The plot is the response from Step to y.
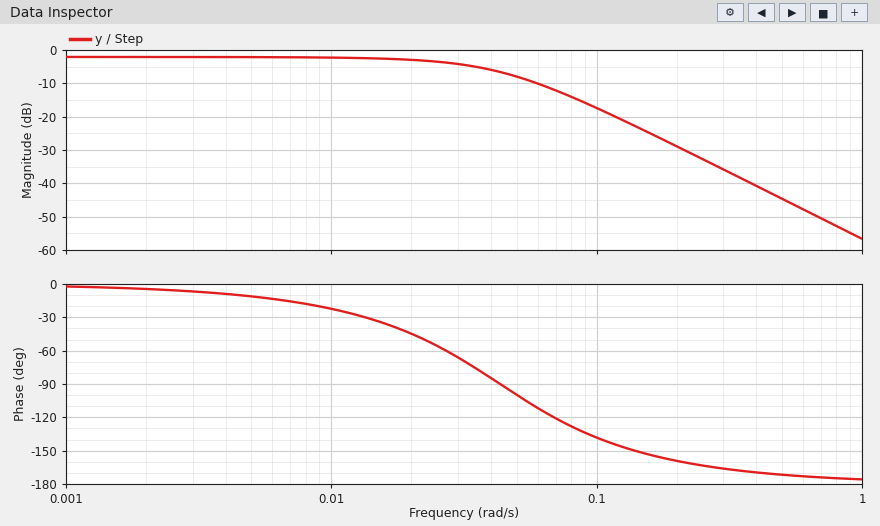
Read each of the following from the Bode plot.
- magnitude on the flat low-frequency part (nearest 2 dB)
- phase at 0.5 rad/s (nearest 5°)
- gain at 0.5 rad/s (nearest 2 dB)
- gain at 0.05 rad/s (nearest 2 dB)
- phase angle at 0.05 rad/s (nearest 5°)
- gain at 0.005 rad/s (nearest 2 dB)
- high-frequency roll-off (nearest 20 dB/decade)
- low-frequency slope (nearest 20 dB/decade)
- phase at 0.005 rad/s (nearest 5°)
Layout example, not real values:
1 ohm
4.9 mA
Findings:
-2 dB
-170°
-44 dB
-8 dB
-100°
-2 dB
-40 dB/decade
0 dB/decade
-10°
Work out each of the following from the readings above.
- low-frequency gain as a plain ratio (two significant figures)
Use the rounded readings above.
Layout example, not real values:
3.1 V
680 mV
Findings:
0.79
